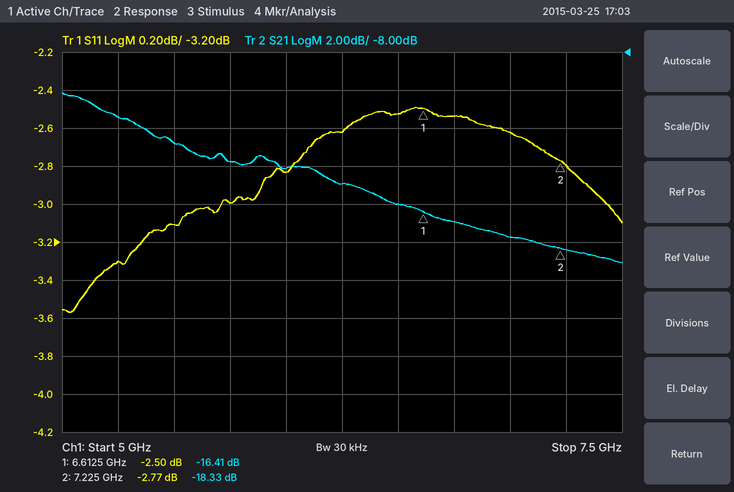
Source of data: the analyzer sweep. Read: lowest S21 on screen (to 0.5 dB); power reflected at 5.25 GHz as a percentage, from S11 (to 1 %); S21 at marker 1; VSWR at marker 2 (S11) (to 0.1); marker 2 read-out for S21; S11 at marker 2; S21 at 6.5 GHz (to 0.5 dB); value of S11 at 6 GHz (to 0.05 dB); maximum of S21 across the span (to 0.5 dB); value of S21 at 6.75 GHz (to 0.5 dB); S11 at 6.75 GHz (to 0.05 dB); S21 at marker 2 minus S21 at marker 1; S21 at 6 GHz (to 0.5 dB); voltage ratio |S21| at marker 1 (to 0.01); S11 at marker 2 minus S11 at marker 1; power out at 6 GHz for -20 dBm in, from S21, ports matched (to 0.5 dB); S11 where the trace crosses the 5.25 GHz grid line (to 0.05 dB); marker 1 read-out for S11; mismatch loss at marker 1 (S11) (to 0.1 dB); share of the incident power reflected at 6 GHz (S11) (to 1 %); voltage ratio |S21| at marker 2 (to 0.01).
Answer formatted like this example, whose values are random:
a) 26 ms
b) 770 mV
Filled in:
a) -19.0 dB
b) 47 %
c) -16.41 dB
d) 6.3
e) -18.33 dB
f) -2.77 dB
g) -16.0 dB
h) -2.85 dB
i) -10.0 dB
j) -17.0 dB
k) -2.55 dB
l) -1.92 dB
m) -14.0 dB
n) 0.15
o) -0.27 dB
p) -34.0 dBm
q) -3.30 dB
r) -2.50 dB
s) 3.6 dB
t) 52 %
u) 0.12
